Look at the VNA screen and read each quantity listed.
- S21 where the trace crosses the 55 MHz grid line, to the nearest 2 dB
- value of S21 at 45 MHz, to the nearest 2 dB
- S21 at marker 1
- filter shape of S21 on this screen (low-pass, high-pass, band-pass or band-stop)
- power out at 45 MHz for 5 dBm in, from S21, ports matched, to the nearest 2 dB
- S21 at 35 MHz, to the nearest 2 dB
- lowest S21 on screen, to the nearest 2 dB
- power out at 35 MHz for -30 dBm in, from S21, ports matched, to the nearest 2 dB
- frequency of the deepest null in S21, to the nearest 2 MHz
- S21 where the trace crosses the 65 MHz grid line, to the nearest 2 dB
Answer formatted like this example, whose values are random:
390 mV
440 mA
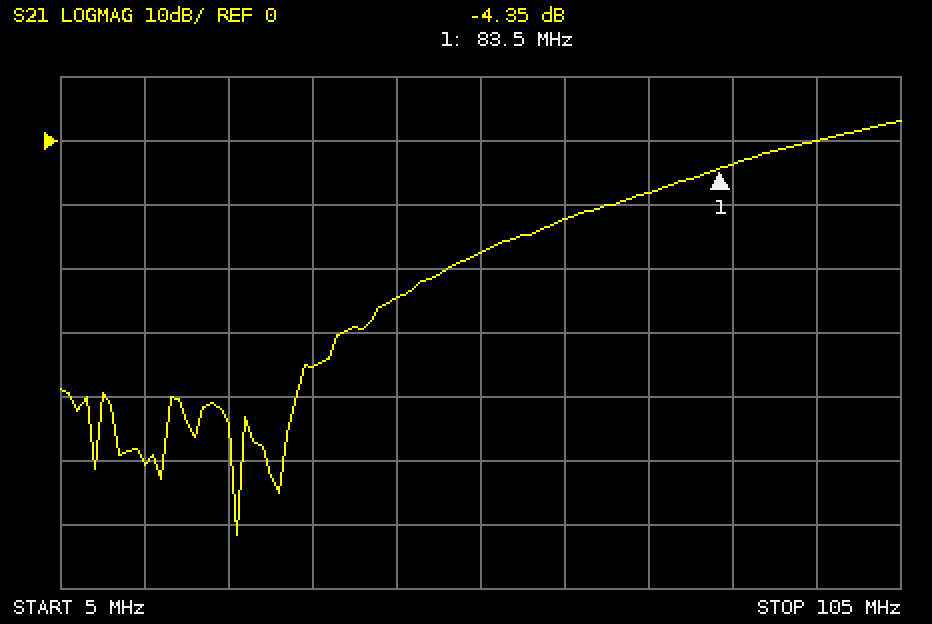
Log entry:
-18 dB
-24 dB
-4.35 dB
high-pass
-20 dBm
-36 dB
-62 dB
-66 dBm
26 MHz
-12 dB
